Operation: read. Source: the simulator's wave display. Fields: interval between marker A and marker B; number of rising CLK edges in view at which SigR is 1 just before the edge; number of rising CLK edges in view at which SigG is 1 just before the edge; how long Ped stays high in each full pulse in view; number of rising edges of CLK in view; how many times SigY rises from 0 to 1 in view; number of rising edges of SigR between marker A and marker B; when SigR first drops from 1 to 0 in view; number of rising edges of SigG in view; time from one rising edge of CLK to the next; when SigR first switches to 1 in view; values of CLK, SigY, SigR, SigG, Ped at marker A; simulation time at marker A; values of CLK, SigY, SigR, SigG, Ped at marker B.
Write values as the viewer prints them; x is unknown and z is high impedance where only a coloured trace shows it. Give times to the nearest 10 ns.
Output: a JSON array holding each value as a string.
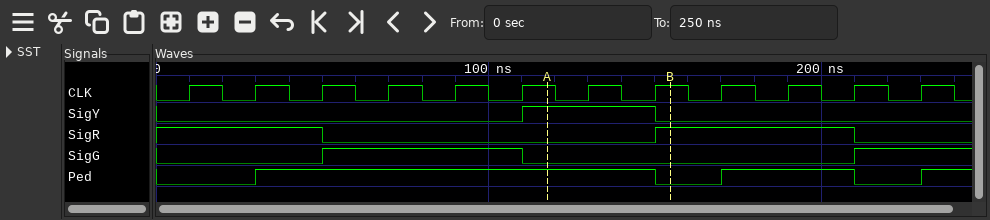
["40 ns", "6", "4", "120 ns, 40 ns", "12", "1", "1", "50 ns", "2", "20 ns", "150 ns", "CLK=1, SigY=1, SigR=0, SigG=0, Ped=1", "120 ns", "CLK=1, SigY=0, SigR=1, SigG=0, Ped=0"]
